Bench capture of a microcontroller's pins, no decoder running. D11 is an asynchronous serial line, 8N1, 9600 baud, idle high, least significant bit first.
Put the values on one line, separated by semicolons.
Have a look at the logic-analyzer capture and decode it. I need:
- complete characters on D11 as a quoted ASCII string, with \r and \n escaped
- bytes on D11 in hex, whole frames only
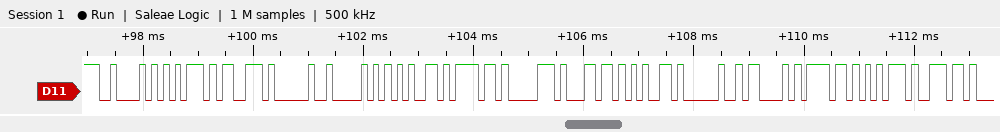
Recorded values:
"Bus People Coun"; 42 75 73 20 50 65 6F 70 6C 65 20 43 6F 75 6E
